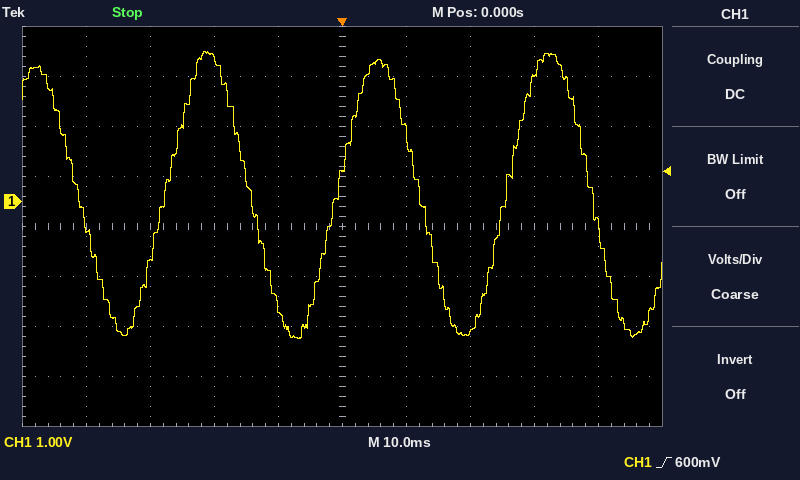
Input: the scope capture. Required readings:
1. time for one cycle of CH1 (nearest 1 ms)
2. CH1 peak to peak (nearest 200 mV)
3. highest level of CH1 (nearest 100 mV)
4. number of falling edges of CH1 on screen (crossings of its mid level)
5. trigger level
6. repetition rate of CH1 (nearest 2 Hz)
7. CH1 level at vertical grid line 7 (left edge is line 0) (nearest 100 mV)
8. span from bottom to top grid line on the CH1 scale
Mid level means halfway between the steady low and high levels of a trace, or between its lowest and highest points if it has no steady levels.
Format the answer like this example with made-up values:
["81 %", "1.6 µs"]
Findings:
["27 ms", "5.8 V", "3.0 V", "4", "600 mV", "38 Hz", "-2.6 V", "8 V"]
